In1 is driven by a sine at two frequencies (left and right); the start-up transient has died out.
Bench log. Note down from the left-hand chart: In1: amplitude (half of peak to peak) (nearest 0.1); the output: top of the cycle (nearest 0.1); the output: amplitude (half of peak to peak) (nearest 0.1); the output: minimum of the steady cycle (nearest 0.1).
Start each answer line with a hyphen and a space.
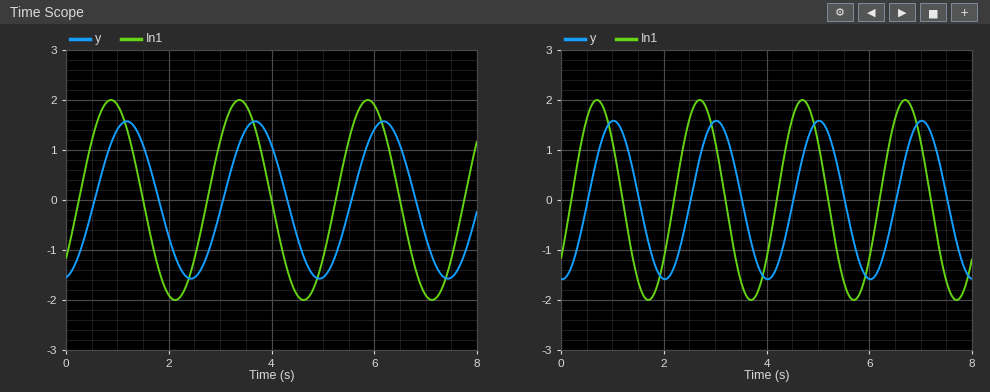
- 2.0
- 1.6
- 1.6
- -1.6
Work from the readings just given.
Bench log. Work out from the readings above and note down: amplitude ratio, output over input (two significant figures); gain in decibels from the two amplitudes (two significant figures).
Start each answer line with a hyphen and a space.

- 0.80
- -1.9 dB
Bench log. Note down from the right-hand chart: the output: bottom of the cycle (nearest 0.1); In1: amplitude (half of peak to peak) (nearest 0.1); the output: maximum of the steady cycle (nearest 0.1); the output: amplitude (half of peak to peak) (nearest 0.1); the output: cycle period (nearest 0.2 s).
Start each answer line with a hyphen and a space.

- -1.6
- 2.0
- 1.6
- 1.6
- 2.0 s
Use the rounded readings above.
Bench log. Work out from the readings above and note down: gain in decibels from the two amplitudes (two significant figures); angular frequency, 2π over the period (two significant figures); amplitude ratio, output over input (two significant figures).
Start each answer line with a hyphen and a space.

- -1.9 dB
- 3.1 rad/s
- 0.80
